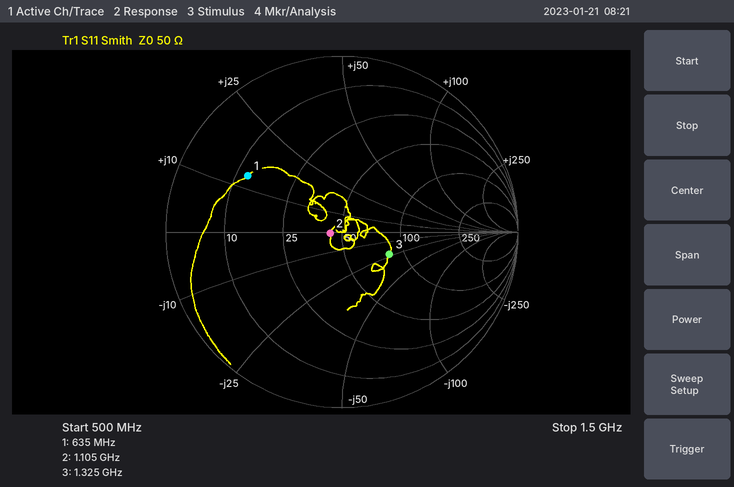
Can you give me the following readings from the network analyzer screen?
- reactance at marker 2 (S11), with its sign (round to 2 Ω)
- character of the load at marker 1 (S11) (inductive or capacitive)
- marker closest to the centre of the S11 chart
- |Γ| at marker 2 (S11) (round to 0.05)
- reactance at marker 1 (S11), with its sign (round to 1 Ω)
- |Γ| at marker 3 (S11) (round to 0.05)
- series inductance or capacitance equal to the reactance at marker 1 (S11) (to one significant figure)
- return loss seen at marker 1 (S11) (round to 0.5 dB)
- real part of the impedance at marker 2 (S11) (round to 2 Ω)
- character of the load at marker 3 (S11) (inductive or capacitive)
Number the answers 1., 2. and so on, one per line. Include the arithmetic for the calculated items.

1. 0 Ω
2. inductive
3. marker 2
4. 0.05
5. +13 Ω
6. 0.30
7. L = 13 Ω/(2π × 635 MHz) ≈ 3 nH
8. 4.0 dB
9. 44 Ω
10. capacitive
